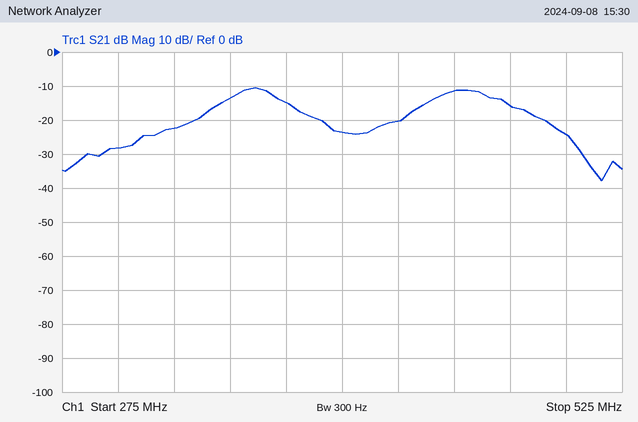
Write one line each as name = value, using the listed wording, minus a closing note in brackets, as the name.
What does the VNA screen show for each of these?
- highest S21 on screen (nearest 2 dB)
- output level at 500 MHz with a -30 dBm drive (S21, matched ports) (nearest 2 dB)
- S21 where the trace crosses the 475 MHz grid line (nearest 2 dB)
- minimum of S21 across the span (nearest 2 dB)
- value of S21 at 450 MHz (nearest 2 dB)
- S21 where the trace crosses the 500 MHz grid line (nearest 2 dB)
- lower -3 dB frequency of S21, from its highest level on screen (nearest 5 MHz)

highest S21 on screen = -10 dB
output level at 500 MHz with a -30 dBm drive (S21, matched ports) = -54 dBm
S21 where the trace crosses the 475 MHz grid line = -16 dB
minimum of S21 across the span = -38 dB
value of S21 at 450 MHz = -12 dB
S21 where the trace crosses the 500 MHz grid line = -24 dB
lower -3 dB frequency of S21, from its highest level on screen = 350 MHz
